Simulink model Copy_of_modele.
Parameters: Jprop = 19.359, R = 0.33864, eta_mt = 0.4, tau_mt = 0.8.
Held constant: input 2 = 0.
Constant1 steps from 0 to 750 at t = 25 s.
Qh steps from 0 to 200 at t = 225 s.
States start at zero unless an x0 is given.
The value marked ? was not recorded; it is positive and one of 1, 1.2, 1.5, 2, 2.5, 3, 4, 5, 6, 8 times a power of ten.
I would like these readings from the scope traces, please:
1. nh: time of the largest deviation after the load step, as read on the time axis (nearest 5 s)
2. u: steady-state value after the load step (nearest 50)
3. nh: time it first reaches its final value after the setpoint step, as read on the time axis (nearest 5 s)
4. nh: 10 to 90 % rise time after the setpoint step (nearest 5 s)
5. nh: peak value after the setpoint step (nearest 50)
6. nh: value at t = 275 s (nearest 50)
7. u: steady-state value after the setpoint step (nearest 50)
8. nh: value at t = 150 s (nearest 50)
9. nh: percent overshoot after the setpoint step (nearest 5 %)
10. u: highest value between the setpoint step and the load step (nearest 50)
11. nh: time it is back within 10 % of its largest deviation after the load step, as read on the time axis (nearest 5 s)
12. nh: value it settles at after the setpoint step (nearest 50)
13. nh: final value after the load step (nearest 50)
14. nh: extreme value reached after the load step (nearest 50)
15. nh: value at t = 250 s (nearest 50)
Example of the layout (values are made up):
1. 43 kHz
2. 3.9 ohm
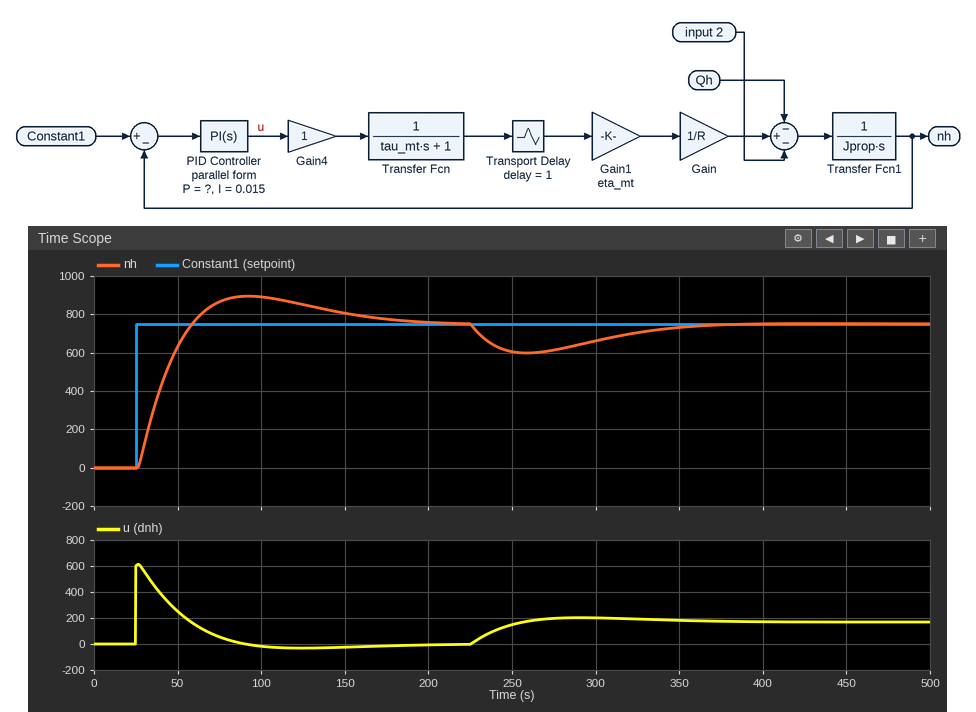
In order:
1. 260 s
2. 150
3. 60 s
4. 25 s
5. 900
6. 600
7. 0
8. 800
9. 20 %
10. 600
11. 355 s
12. 750
13. 750
14. 600
15. 600
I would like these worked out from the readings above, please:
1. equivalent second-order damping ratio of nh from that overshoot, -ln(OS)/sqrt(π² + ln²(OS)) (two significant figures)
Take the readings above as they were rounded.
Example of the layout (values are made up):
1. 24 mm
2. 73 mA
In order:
1. 0.46
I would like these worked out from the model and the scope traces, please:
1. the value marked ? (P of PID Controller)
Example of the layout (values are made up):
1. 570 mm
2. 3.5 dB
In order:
1. 0.8
